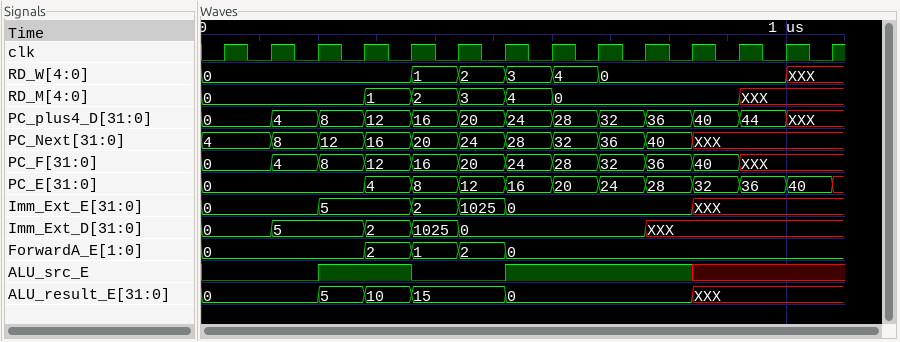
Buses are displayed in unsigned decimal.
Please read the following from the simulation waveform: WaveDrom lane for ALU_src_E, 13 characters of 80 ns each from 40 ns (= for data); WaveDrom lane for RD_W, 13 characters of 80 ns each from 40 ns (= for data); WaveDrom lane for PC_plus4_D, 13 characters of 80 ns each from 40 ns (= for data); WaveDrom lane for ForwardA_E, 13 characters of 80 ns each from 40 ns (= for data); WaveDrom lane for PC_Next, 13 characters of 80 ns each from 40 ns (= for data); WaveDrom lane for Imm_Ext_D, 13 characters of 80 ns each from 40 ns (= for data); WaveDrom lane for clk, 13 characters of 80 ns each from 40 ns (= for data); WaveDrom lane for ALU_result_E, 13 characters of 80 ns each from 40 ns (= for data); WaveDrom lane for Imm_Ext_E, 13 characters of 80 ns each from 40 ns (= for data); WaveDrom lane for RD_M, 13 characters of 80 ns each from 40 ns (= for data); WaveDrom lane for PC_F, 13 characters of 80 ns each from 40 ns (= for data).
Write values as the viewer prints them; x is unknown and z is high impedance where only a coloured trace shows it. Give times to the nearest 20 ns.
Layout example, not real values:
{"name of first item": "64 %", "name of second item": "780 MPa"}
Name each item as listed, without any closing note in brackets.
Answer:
{"WaveDrom lane for ALU_src_E, 13 characters of 80 ns each from 40 ns": "{name: 'ALU_src_E', wave: '0.1.0.1...x..'}", "WaveDrom lane for RD_W, 13 characters of 80 ns each from 40 ns": "{name: 'RD_W', wave: '=...=====...x', data: '0 1 2 3 4 0'}", "WaveDrom lane for PC_plus4_D, 13 characters of 80 ns each from 40 ns": "{name: 'PC_plus4_D', wave: '============x', data: '0 4 8 12 16 20 24 28 32 36 40 44'}", "WaveDrom lane for ForwardA_E, 13 characters of 80 ns each from 40 ns": "{name: 'ForwardA_E', wave: '=..====......', data: '0 2 1 2 0'}", "WaveDrom lane for PC_Next, 13 characters of 80 ns each from 40 ns": "{name: 'PC_Next', wave: '==========x..', data: '4 8 12 16 20 24 28 32 36 40'}", "WaveDrom lane for Imm_Ext_D, 13 characters of 80 ns each from 40 ns": "{name: 'Imm_Ext_D', wave: '==.===...x...', data: '0 5 2 1025 0'}", "WaveDrom lane for clk, 13 characters of 80 ns each from 40 ns": "{name: 'clk', wave: 'p............'}", "WaveDrom lane for ALU_result_E, 13 characters of 80 ns each from 40 ns": "{name: 'ALU_result_E', wave: '=.===.=...x..', data: '0 5 10 15 0'}", "WaveDrom lane for Imm_Ext_E, 13 characters of 80 ns each from 40 ns": "{name: 'Imm_Ext_E', wave: '=.=.===...x..', data: '0 5 2 1025 0'}", "WaveDrom lane for RD_M, 13 characters of 80 ns each from 40 ns": "{name: 'RD_M', wave: '=..=====...x.', data: '0 1 2 3 4 0'}", "WaveDrom lane for PC_F, 13 characters of 80 ns each from 40 ns": "{name: 'PC_F', wave: '===========x.', data: '0 4 8 12 16 20 24 28 32 36 40'}"}
